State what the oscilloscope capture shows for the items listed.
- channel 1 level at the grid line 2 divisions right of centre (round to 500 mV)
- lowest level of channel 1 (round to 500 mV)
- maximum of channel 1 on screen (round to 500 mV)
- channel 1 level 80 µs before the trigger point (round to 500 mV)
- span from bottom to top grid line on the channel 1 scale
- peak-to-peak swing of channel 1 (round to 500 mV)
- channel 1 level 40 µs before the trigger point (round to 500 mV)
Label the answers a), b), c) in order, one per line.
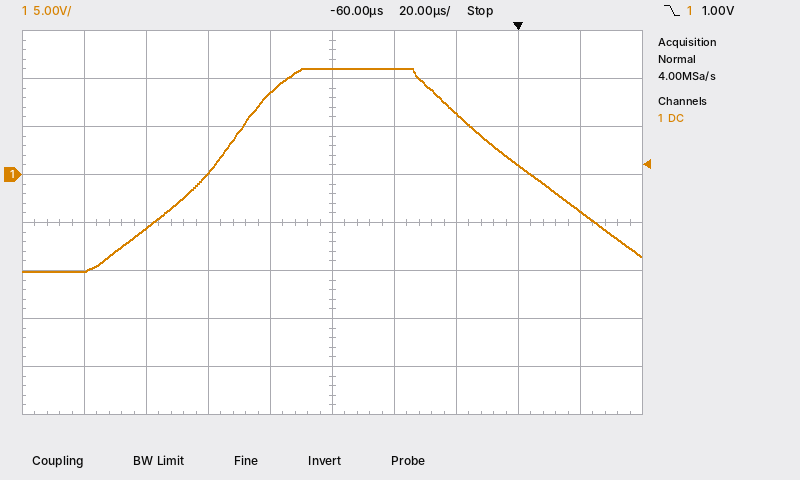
a) 6.5 V
b) -10.0 V
c) 11.0 V
d) 8.5 V
e) 40 V
f) 21.0 V
g) 11.0 V
